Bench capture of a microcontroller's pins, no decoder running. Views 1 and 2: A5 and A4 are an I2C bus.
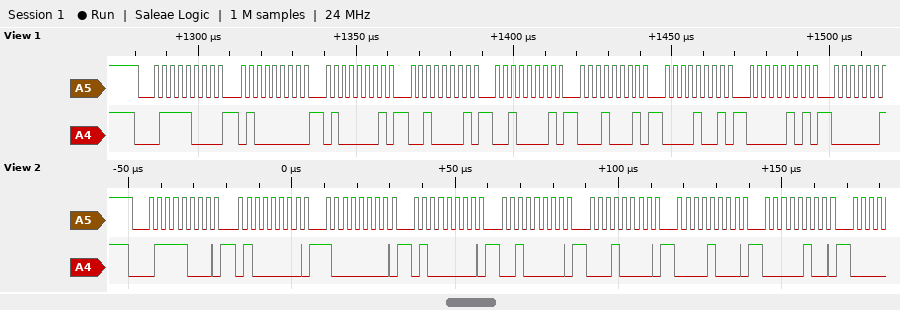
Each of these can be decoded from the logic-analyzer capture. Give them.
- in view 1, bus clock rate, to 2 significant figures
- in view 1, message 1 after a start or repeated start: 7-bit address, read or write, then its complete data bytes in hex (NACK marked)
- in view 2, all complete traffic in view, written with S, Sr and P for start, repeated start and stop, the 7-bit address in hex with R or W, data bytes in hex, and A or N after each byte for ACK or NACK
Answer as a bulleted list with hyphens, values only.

- 400 kHz
- 0x3C write: 40 41 21 21 11 09 05
- S 3CW A 40 A 80 A 40 A 20 A 10 A 08 A 04 A
